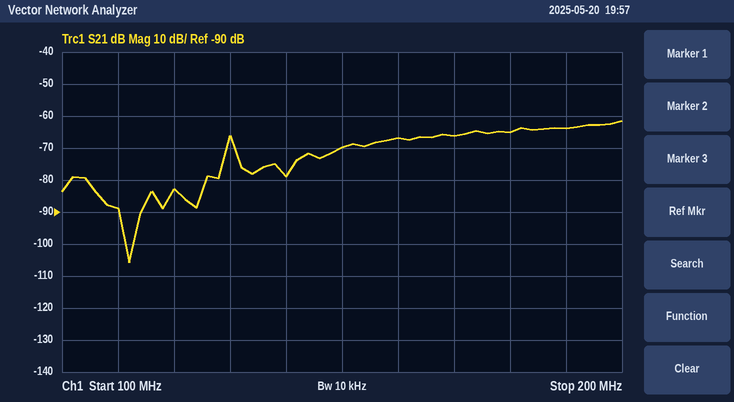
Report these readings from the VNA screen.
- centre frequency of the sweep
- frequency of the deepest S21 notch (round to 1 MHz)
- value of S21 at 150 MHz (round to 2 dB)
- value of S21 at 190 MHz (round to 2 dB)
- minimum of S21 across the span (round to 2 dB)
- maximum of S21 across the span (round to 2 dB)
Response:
150 MHz
112 MHz
-70 dB
-64 dB
-106 dB
-62 dB
